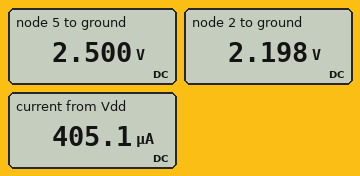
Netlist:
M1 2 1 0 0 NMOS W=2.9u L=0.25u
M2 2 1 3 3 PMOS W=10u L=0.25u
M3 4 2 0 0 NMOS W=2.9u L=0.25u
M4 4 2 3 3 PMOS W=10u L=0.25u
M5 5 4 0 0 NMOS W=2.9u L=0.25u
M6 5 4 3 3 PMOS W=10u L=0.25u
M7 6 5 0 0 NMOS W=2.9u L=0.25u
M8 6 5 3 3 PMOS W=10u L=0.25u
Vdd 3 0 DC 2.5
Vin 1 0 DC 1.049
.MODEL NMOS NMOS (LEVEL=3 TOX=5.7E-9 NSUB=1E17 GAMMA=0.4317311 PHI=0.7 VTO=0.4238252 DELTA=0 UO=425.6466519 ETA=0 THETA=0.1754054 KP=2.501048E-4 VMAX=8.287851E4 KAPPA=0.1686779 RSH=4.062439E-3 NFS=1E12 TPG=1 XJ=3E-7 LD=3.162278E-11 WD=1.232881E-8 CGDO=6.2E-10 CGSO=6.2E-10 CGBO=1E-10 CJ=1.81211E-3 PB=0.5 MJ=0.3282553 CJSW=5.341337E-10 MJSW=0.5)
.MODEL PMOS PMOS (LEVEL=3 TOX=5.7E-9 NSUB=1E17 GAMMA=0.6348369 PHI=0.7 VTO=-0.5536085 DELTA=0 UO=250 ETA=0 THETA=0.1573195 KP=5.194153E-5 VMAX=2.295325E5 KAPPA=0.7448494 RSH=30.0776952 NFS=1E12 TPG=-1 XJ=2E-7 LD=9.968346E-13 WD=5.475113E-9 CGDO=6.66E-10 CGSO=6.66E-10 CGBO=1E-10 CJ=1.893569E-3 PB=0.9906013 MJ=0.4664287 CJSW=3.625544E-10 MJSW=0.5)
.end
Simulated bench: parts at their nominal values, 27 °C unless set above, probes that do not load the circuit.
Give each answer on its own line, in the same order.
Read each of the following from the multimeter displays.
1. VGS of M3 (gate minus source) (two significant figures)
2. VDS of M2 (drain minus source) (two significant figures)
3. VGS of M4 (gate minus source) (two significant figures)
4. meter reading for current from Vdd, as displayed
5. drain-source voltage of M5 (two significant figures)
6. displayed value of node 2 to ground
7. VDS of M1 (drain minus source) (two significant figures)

2.2 V
-300 mV
-300 mV
405.1 µA
2.5 V
2.198 V
2.2 V
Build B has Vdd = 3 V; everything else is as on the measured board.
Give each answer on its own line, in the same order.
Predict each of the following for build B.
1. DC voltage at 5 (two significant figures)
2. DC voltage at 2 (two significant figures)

3.0 V
2.8 V
